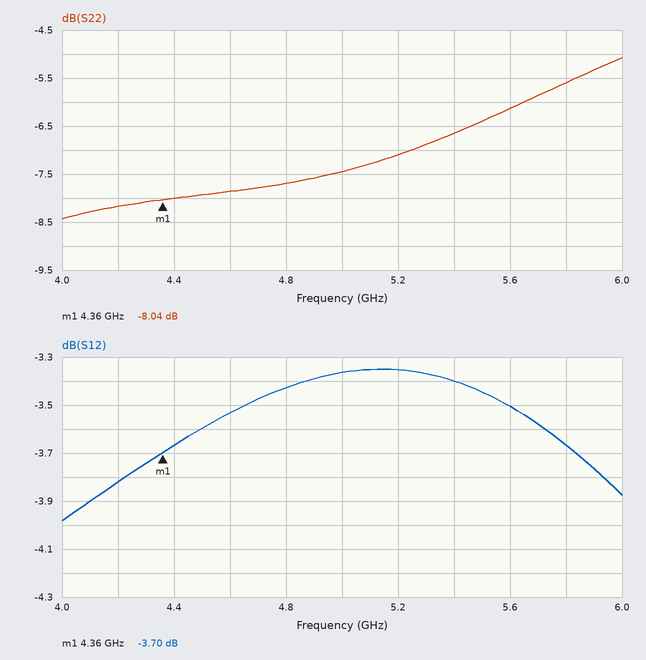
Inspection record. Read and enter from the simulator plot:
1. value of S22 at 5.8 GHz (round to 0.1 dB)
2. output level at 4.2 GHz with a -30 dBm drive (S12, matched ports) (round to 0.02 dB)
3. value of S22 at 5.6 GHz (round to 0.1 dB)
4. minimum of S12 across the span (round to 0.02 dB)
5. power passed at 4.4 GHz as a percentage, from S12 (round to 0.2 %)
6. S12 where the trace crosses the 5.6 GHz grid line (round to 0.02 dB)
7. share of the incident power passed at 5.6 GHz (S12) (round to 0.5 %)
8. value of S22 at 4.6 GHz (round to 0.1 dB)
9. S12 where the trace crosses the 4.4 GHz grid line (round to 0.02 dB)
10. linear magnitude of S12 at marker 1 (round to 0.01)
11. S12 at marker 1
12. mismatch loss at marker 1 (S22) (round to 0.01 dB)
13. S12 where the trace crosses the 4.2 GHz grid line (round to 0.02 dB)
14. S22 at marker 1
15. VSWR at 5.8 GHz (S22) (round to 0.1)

-5.6 dB
-33.82 dBm
-6.1 dB
-3.98 dB
43.0 %
-3.50 dB
44.5 %
-7.9 dB
-3.66 dB
0.65
-3.70 dB
0.74 dB
-3.82 dB
-8.04 dB
3.2
